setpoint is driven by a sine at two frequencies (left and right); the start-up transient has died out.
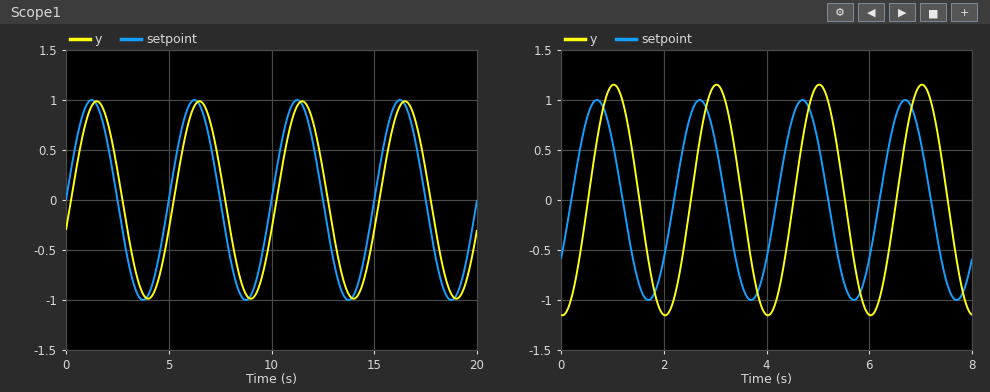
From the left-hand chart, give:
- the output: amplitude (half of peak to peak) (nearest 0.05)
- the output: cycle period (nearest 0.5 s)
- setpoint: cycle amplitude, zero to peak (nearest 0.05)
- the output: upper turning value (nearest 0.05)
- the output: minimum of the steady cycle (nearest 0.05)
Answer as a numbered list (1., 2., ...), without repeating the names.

1. 1.00
2. 5.0 s
3. 1.00
4. 1.00
5. -1.00
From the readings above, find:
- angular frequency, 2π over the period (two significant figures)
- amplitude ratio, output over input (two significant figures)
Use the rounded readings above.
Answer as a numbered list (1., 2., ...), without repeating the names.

1. 1.3 rad/s
2. 1.0
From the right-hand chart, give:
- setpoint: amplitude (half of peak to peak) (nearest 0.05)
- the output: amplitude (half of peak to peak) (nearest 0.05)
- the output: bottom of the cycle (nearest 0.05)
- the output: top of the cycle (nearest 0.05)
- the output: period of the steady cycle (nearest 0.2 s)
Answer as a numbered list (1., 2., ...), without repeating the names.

1. 1.00
2. 1.15
3. -1.15
4. 1.15
5. 2.0 s
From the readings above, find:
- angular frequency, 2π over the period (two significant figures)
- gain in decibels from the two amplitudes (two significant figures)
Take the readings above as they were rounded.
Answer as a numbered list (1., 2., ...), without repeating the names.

1. 3.1 rad/s
2. 1.2 dB
